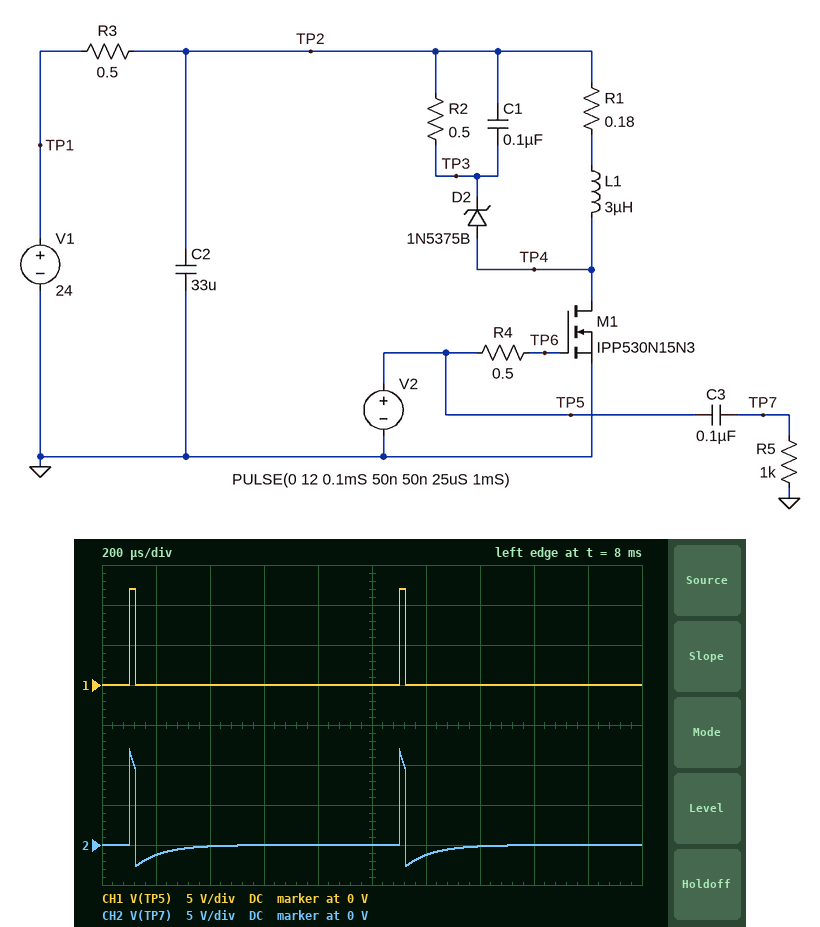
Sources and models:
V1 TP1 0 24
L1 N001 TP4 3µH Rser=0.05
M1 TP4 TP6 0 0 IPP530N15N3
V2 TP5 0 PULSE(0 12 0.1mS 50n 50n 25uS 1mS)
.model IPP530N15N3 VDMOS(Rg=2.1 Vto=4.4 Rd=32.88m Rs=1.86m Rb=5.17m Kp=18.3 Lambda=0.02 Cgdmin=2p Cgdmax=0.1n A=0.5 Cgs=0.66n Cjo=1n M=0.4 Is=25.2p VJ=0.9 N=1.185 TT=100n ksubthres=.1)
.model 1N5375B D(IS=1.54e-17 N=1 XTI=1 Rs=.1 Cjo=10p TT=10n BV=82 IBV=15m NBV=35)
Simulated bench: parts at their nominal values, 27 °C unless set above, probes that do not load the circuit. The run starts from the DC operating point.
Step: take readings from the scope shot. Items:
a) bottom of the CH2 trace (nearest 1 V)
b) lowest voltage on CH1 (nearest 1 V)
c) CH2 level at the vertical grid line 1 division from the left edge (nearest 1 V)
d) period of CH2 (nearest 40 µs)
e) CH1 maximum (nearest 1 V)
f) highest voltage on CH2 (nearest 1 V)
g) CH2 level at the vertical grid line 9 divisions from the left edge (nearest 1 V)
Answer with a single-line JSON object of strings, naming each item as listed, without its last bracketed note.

{"bottom of the CH2 trace": "-3 V", "lowest voltage on CH1": "0 V", "CH2 level at the vertical grid line 1 division from the left edge": "-1 V", "period of CH2": "1.00 ms", "CH1 maximum": "12 V", "highest voltage on CH2": "12 V", "CH2 level at the vertical grid line 9 divisions from the left edge": "0 V"}
